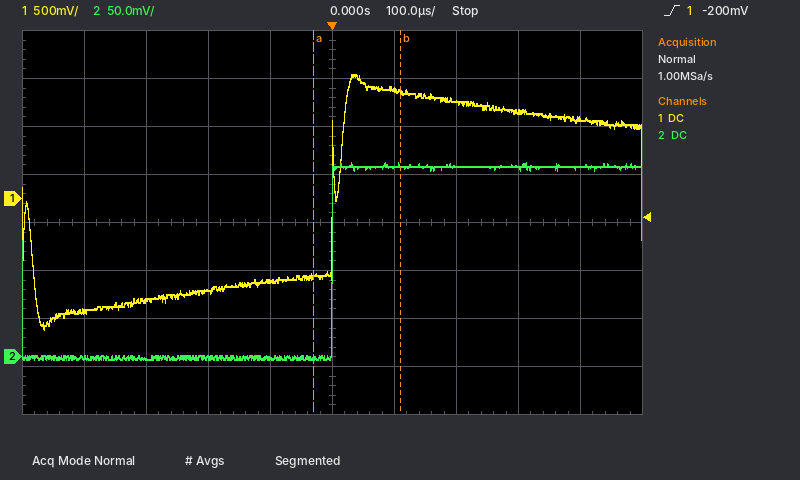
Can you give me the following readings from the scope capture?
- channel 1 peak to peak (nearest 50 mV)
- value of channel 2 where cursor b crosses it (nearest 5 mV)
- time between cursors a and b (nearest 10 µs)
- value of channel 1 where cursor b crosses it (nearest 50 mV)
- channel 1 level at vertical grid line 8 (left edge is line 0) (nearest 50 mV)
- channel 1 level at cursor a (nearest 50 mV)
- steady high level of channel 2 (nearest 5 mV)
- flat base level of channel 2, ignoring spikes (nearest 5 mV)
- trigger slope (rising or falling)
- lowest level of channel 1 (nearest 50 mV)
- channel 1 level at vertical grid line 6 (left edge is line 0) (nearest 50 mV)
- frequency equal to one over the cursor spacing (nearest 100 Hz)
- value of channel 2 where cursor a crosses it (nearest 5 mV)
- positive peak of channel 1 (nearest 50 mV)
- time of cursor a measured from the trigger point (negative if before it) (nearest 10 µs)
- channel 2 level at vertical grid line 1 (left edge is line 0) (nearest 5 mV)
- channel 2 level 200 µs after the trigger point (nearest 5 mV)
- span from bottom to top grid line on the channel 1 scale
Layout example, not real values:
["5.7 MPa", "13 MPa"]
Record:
["2.65 V", "200 mV", "140 µs", "1.10 V", "900 mV", "-800 mV", "200 mV", "0 mV", "rising", "-1.35 V", "1.15 V", "7.1 kHz", "0 mV", "1.30 V", "-30 µs", "0 mV", "200 mV", "4 V"]
